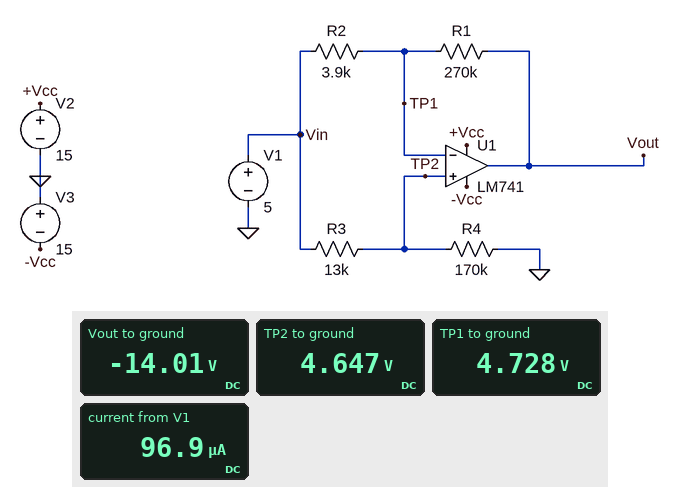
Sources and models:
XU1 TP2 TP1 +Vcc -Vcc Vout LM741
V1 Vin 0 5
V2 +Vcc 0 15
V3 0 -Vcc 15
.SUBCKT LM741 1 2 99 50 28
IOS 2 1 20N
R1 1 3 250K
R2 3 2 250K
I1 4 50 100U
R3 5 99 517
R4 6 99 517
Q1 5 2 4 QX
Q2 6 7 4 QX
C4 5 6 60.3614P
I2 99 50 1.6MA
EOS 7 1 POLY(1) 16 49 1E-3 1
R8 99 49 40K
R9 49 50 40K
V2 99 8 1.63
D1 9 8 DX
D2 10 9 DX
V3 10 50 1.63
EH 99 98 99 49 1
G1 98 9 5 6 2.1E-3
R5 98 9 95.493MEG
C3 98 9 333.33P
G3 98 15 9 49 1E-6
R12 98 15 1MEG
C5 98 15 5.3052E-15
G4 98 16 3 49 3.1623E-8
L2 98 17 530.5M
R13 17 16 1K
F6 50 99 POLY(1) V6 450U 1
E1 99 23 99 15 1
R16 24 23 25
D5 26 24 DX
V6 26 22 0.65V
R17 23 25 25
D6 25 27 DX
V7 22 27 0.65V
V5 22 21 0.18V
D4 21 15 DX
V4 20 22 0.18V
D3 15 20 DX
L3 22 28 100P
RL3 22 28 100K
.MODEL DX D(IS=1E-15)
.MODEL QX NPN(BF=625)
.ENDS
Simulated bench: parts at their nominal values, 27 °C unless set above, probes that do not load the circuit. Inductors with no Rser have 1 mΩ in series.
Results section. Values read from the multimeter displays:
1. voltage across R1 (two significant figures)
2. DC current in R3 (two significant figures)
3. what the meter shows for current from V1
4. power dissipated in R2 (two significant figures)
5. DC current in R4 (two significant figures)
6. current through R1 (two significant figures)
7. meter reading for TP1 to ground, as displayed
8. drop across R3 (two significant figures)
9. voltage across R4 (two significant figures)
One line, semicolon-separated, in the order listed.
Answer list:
19 V; 27 µA; 96.9 µA; 19 µW; 27 µA; 69 µA; 4.728 V; 350 mV; 4.6 V
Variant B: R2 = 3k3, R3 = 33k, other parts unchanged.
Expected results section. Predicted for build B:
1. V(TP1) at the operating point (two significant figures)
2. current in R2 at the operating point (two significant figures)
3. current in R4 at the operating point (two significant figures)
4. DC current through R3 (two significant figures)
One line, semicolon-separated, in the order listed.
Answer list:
4.8 V; 71 µA; 25 µA; 24 µA
